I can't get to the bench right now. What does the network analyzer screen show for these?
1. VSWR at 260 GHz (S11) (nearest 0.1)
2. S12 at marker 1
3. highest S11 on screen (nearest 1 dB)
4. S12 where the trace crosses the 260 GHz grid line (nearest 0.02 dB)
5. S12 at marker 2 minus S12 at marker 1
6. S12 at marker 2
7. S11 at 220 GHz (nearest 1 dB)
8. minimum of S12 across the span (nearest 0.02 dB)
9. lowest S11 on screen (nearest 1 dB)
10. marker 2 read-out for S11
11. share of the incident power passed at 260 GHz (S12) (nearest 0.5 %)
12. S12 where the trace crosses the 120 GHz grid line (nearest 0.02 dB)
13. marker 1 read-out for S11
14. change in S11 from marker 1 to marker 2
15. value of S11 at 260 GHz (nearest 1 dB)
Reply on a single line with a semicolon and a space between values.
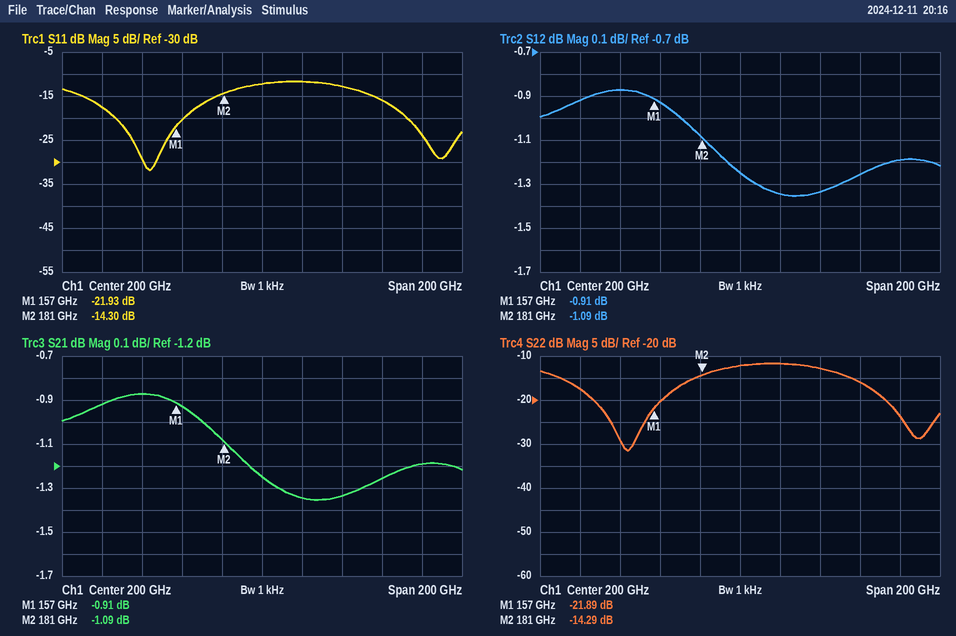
1.4; -0.91 dB; -12 dB; -1.26 dB; -0.18 dB; -1.09 dB; -12 dB; -1.36 dB; -32 dB; -14.30 dB; 75.0 %; -0.92 dB; -21.93 dB; 7.63 dB; -16 dB
